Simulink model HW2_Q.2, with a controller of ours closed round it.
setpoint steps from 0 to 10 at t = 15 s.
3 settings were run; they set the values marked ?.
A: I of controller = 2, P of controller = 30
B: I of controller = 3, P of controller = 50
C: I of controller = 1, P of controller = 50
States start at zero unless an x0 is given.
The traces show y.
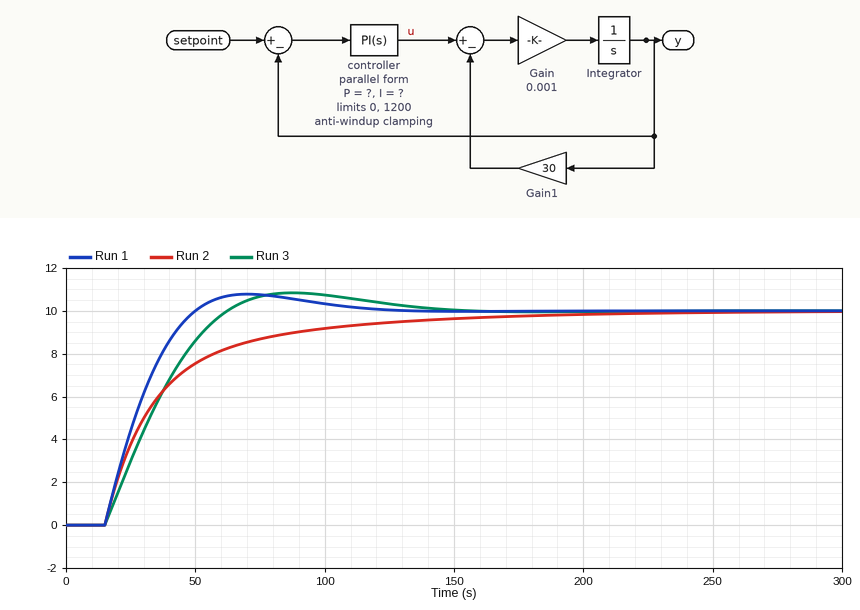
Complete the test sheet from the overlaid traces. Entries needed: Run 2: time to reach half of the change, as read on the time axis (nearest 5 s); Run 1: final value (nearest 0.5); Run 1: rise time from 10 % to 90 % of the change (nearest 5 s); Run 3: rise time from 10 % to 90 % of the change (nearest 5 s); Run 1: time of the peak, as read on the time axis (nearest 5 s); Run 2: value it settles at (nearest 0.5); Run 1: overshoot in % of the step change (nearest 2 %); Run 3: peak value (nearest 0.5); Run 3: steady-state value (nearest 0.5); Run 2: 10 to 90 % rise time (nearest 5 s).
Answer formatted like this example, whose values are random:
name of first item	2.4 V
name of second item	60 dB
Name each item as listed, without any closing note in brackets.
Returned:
Run 2: time to reach half of the change, as read on the time axis	30 s
Run 1: final value	10.0
Run 1: rise time from 10 % to 90 % of the change	25 s
Run 3: rise time from 10 % to 90 % of the change	35 s
Run 1: time of the peak, as read on the time axis	70 s
Run 2: value it settles at	10.0
Run 1: overshoot in % of the step change	8 %
Run 3: peak value	11.0
Run 3: steady-state value	10.0
Run 2: 10 to 90 % rise time	70 s
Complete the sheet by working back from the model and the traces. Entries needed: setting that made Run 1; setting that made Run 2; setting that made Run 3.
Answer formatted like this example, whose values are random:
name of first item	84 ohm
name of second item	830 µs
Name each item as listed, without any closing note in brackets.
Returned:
setting that made Run 1	B
setting that made Run 2	C
setting that made Run 3	A
